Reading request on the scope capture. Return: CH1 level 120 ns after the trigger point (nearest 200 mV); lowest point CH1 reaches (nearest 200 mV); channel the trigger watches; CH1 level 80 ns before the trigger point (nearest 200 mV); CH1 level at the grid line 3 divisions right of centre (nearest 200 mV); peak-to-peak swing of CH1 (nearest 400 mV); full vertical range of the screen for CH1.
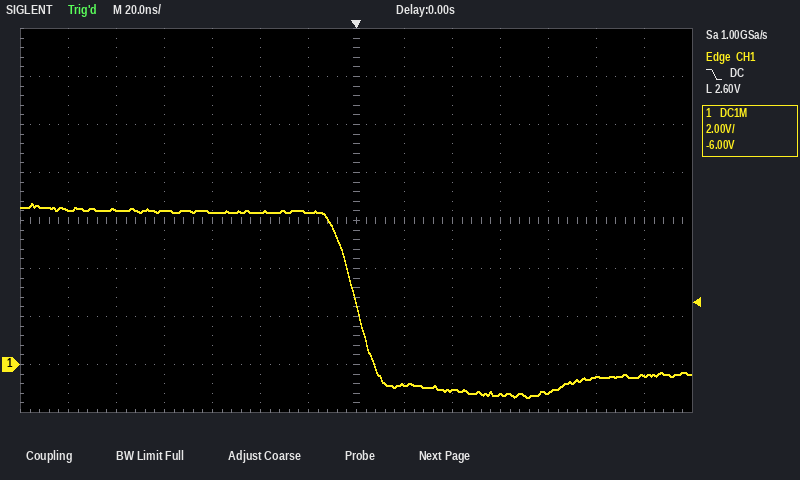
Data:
-400 mV
-1.4 V
CH1
6.4 V
-1.2 V
8.0 V
16 V
